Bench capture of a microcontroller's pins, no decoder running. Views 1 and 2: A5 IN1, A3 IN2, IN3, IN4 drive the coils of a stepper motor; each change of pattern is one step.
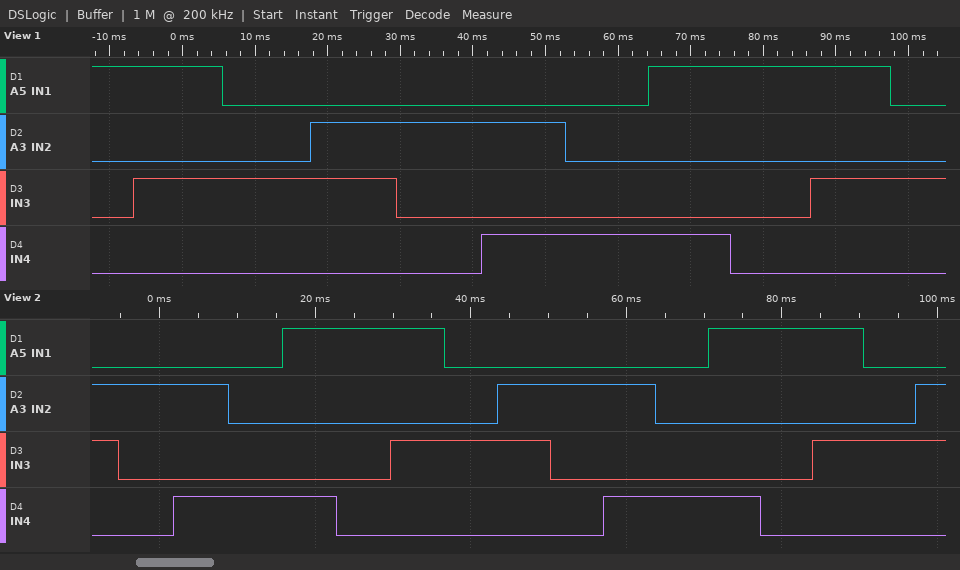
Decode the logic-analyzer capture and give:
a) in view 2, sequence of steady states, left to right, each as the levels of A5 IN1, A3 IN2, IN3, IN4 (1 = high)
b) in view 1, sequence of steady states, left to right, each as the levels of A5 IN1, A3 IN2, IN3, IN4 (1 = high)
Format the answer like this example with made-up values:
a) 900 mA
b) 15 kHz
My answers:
a) 0110 0100 0101 0001 1001 1000 1010 0010 0110 0100 0101 0001 1001 1000 1010 0010 0110
b) 1000 1010 0010 0110 0100 0101 0001 1001 1000 1010 0010
